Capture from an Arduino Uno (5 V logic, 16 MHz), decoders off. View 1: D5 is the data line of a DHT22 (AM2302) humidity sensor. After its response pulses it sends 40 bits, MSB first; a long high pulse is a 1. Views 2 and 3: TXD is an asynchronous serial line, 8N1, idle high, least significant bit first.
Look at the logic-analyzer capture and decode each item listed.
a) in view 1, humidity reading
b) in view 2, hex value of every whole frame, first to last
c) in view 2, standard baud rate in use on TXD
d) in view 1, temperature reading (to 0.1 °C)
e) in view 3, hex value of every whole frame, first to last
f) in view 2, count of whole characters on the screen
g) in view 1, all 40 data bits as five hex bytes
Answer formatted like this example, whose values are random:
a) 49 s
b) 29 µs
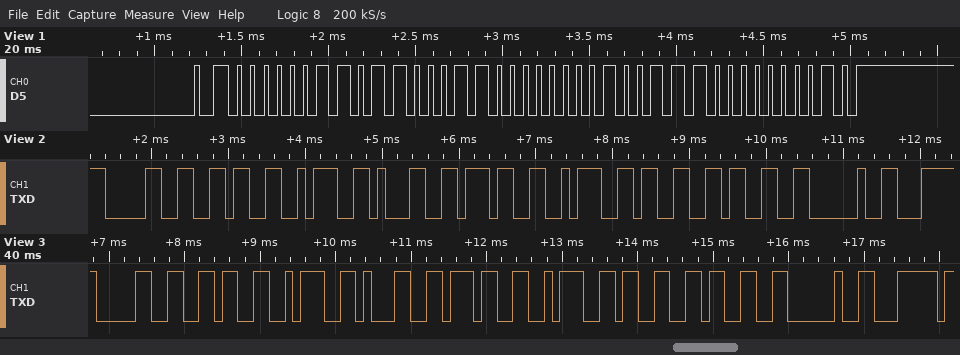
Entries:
a) 86.7 %
b) 0x30 0x36 0x3A 0x31 0x37 0x3A 0x33 0x33 0x20
c) 9600 baud
d) 15.6 °C
e) 30 36 3A 31 37 3A 33 33 20 7C
f) 9
g) 03 63 00 9C 02
